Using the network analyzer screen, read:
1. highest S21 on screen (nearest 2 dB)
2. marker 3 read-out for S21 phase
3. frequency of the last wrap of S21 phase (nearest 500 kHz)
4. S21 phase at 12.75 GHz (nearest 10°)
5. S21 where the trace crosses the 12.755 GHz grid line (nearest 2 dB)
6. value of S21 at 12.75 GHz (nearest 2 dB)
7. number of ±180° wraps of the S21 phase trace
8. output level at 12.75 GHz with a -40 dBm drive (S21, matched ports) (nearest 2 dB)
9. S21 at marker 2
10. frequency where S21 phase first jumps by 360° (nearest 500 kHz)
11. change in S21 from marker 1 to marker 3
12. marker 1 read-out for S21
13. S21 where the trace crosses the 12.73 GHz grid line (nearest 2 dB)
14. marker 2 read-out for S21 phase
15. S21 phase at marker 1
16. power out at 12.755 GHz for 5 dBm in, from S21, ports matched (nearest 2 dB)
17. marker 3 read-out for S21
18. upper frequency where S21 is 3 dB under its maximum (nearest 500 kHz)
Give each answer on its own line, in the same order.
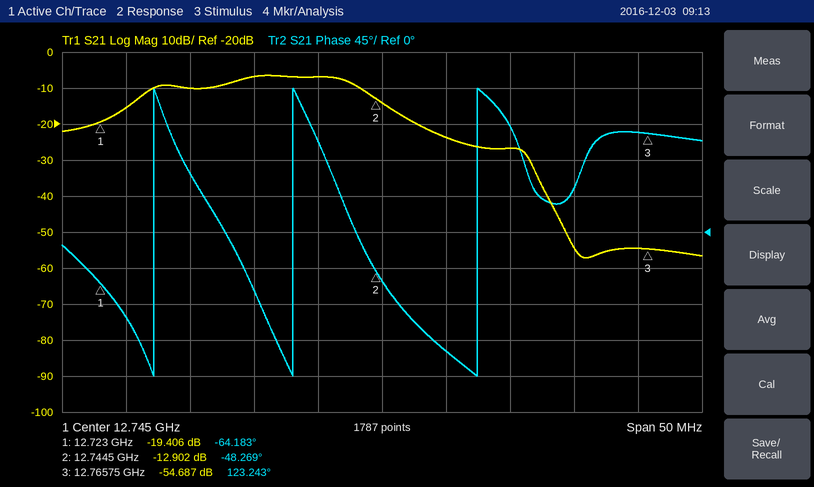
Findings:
-6 dB
123.243°
12.7525 GHz
-150°
-26 dB
-24 dB
3
-64 dBm
-12.902 dB
12.7270 GHz
-35.281 dB
-19.406 dB
-10 dB
-48.269°
-64.183°
-22 dBm
-54.687 dB
12.7430 GHz
